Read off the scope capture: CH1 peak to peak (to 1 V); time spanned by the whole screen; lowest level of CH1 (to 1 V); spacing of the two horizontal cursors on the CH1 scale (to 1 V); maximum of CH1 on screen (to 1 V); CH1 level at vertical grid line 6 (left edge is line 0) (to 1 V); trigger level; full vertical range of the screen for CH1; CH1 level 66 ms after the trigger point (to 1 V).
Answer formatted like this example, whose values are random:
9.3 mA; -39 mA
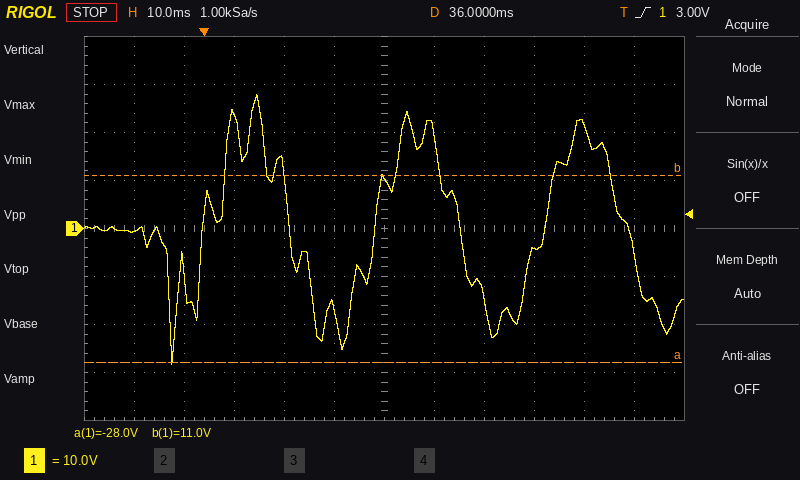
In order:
56 V; 120 ms; -28 V; 39 V; 28 V; 10 V; 3.00 V; 80 V; -4 V
